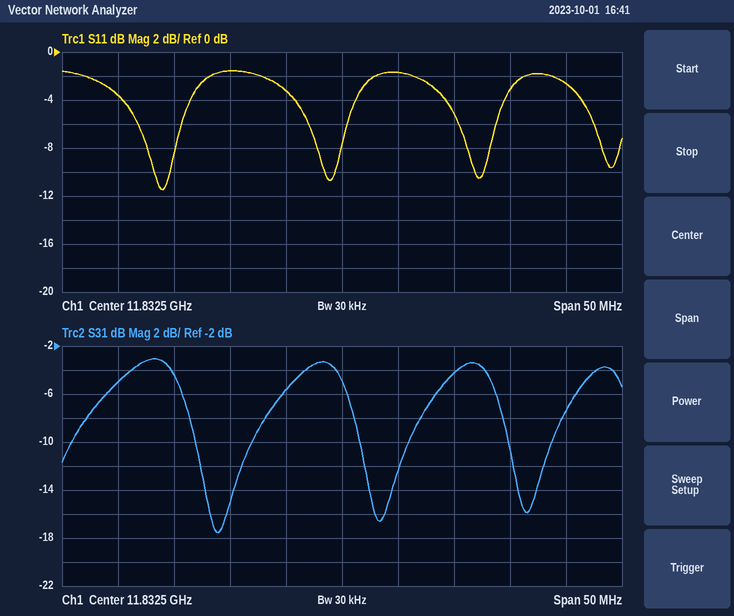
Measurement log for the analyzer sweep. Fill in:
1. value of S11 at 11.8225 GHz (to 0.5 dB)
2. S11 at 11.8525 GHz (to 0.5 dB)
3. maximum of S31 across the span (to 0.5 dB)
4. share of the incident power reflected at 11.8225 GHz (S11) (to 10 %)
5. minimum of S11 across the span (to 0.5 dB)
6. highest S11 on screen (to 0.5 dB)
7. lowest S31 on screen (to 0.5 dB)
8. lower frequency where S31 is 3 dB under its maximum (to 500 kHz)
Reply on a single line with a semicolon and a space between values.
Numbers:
-1.5 dB; -2.5 dB; -3.0 dB; 70 %; -11.5 dB; -1.5 dB; -17.5 dB; 11.8115 GHz
